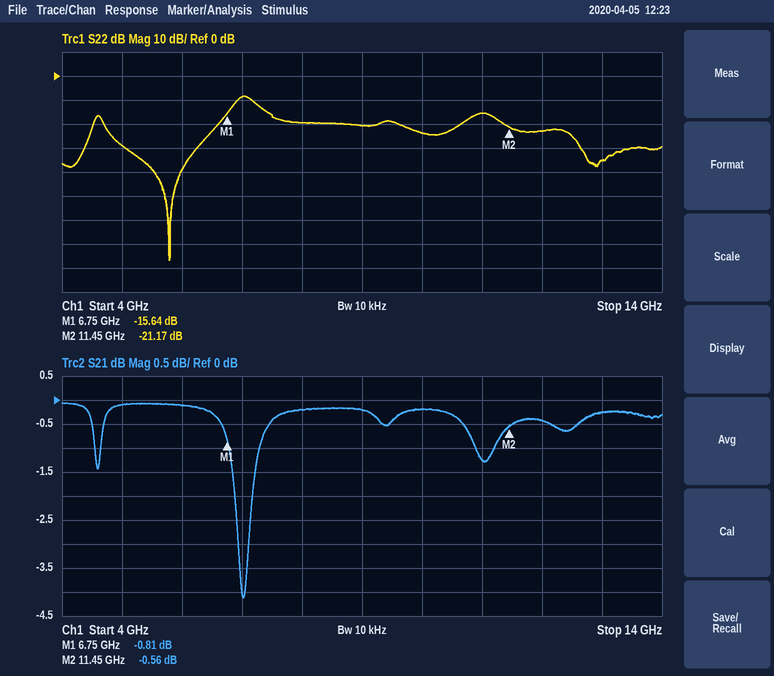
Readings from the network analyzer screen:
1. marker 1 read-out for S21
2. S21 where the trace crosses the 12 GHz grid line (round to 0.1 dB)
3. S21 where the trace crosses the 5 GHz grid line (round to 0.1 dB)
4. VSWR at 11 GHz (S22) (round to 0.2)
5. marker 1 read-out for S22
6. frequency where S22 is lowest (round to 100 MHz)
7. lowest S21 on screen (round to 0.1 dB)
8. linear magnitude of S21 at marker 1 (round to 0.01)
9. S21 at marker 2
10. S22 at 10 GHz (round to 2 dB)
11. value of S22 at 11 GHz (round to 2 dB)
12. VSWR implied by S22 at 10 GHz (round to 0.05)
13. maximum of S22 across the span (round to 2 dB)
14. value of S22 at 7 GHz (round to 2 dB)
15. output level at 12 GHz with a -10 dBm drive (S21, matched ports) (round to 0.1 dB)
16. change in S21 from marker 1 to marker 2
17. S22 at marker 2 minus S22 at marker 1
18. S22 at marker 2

-0.81 dB
-0.4 dB
-0.1 dB
1.4
-15.64 dB
5.8 GHz
-4.1 dB
0.91
-0.56 dB
-24 dB
-16 dB
1.15
-8 dB
-8 dB
-10.4 dBm
0.25 dB
-5.53 dB
-21.17 dB
